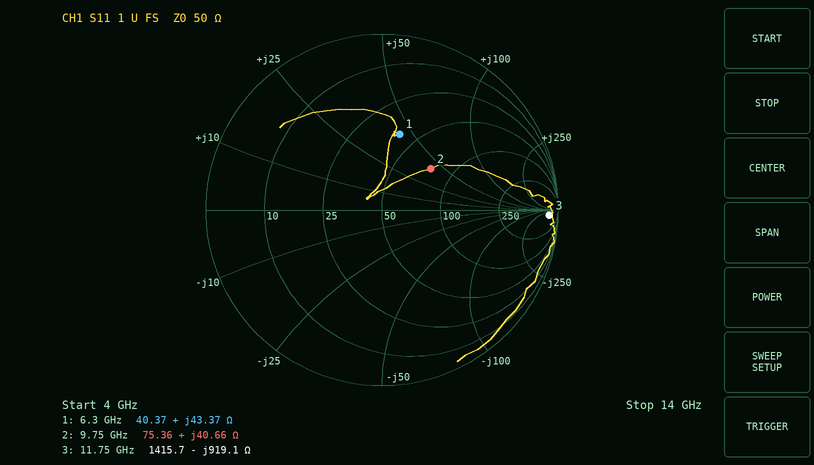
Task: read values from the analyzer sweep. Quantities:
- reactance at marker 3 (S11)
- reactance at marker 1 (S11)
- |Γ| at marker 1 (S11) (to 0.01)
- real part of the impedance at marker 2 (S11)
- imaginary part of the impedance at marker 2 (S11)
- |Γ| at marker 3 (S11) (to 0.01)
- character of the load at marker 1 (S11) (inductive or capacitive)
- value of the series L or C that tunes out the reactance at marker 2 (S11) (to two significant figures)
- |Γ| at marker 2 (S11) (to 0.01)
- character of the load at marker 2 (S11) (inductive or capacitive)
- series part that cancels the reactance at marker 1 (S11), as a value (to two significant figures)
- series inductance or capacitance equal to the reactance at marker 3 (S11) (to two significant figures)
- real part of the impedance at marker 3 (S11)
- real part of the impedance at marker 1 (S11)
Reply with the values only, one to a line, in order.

-919.1 Ω
+43.37 Ω
0.44
75.36 Ω
+40.66 Ω
0.95
inductive
400 fF
0.36
inductive
580 fF
15 fF
1415.7 Ω
40.37 Ω
